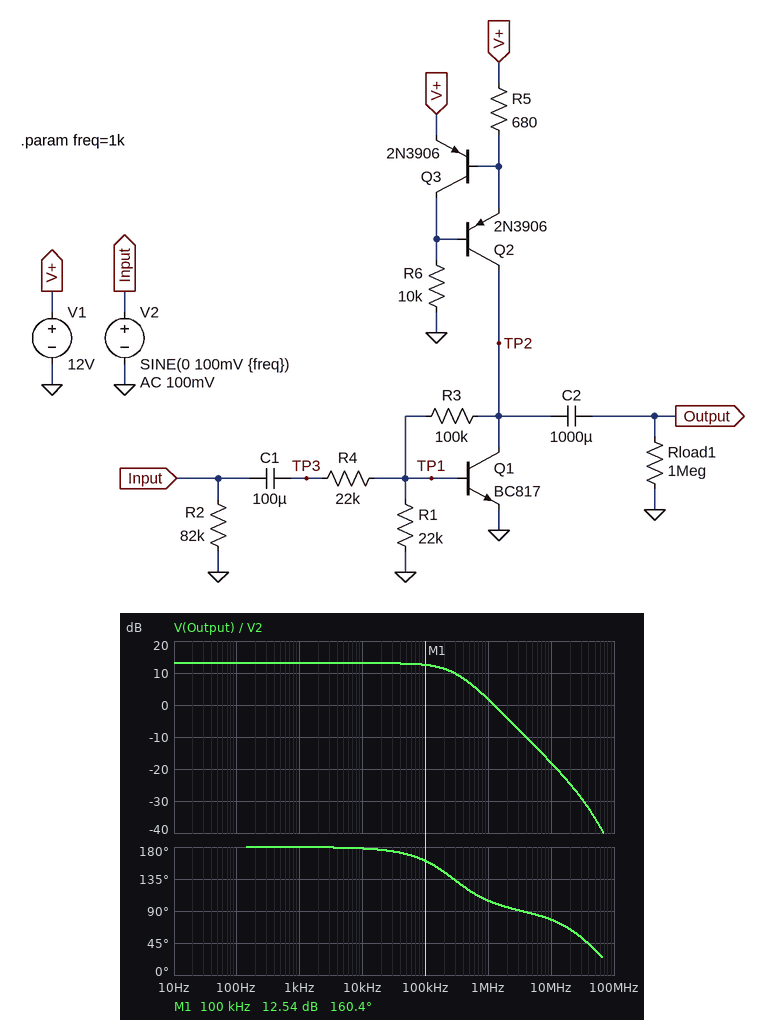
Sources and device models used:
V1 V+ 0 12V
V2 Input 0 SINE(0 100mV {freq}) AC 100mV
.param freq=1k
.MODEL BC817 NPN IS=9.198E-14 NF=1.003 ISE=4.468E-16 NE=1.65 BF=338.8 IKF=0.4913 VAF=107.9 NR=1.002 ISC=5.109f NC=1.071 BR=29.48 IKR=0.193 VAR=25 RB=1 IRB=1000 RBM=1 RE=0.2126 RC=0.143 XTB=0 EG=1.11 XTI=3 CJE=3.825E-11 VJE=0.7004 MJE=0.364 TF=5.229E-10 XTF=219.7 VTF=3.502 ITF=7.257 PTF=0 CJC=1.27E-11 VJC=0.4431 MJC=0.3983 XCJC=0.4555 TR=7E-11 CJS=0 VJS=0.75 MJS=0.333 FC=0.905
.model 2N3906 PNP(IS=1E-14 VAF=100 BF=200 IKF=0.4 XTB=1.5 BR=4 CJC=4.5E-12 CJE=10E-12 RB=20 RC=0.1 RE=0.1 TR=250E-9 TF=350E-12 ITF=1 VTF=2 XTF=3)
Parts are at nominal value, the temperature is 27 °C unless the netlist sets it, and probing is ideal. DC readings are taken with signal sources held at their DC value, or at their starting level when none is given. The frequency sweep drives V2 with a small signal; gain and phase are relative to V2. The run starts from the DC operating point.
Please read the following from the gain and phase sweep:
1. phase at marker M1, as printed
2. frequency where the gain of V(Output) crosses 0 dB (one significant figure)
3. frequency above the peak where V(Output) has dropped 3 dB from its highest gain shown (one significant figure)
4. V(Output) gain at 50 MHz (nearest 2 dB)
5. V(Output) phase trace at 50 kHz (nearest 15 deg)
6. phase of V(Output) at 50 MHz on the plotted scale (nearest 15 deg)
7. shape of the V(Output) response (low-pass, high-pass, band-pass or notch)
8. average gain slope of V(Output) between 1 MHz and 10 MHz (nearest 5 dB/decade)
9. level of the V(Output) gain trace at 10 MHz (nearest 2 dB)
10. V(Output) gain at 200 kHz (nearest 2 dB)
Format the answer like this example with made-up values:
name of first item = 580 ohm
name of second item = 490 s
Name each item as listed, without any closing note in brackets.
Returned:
phase at marker M1, as printed = 160.4 deg
frequency where the gain of V(Output) crosses 0 dB = 1 MHz
frequency above the peak where V(Output) has dropped 3 dB from its highest gain shown = 300 kHz
V(Output) gain at 50 MHz = -36 dB
V(Output) phase trace at 50 kHz = 165 deg
phase of V(Output) at 50 MHz on the plotted scale = 30 deg
shape of the V(Output) response = low-pass
average gain slope of V(Output) between 1 MHz and 10 MHz = -20 dB/decade
level of the V(Output) gain trace at 10 MHz = -18 dB
V(Output) gain at 200 kHz = 12 dB
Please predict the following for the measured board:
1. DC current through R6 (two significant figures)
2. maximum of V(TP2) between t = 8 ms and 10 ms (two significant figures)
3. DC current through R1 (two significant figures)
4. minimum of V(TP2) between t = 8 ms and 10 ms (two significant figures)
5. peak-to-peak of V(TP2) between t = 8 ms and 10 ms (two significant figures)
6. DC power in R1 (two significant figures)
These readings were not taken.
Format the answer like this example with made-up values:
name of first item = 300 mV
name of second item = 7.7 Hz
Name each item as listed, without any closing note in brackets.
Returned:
DC current through R6 = 1.1 mA
maximum of V(TP2) between t = 8 ms and 10 ms = 4.0 V
DC current through R1 = 27 µA
minimum of V(TP2) between t = 8 ms and 10 ms = 3.1 V
peak-to-peak of V(TP2) between t = 8 ms and 10 ms = 900 mV
DC power in R1 = 16 µW
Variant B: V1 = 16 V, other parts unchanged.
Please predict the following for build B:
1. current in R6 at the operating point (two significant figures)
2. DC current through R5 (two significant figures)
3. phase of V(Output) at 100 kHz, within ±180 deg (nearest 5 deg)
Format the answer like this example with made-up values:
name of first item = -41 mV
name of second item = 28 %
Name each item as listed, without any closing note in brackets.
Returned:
current in R6 at the operating point = 1.5 mA
DC current through R5 = 980 µA
phase of V(Output) at 100 kHz, within ±180 deg = 160 deg
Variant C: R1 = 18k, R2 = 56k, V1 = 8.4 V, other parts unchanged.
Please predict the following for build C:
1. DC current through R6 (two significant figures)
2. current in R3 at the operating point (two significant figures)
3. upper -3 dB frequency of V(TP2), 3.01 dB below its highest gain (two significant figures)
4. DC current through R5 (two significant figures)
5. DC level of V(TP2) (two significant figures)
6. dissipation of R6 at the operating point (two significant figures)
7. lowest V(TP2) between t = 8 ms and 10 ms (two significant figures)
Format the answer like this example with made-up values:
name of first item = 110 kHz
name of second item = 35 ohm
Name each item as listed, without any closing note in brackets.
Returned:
DC current through R6 = 710 µA
current in R3 at the operating point = 36 µA
upper -3 dB frequency of V(TP2), 3.01 dB below its highest gain = 300 kHz
DC current through R5 = 950 µA
DC level of V(TP2) = 4.2 V
dissipation of R6 at the operating point = 5.0 mW
lowest V(TP2) between t = 8 ms and 10 ms = 3.7 V
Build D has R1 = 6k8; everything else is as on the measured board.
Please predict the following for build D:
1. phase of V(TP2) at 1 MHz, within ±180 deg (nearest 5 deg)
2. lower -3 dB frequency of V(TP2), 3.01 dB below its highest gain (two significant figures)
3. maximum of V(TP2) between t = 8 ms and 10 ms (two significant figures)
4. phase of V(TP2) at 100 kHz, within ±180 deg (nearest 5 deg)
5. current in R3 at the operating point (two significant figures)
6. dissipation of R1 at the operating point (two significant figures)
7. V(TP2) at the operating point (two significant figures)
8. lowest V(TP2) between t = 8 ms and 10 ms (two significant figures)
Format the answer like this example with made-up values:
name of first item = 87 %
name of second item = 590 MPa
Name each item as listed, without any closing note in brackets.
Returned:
phase of V(TP2) at 1 MHz, within ±180 deg = 110 deg
lower -3 dB frequency of V(TP2), 3.01 dB below its highest gain = 72 mHz
maximum of V(TP2) between t = 8 ms and 10 ms = 10 V
phase of V(TP2) at 100 kHz, within ±180 deg = 165 deg
current in R3 at the operating point = 90 µA
dissipation of R1 at the operating point = 52 µW
V(TP2) at the operating point = 9.6 V
lowest V(TP2) between t = 8 ms and 10 ms = 9.1 V
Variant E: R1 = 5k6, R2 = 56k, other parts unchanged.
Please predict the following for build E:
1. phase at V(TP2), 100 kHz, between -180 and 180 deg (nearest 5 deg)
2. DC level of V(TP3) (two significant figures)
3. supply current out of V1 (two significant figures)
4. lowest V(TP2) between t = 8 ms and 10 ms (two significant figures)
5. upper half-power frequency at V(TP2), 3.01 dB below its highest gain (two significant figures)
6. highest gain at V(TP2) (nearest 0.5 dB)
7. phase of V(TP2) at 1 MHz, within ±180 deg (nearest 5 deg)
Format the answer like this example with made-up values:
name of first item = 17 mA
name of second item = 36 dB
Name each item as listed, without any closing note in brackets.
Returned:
phase at V(TP2), 100 kHz, between -180 and 180 deg = 145 deg
DC level of V(TP3) = 590 mV
supply current out of V1 = 1.9 mA
lowest V(TP2) between t = 8 ms and 10 ms = 11 V
upper half-power frequency at V(TP2), 3.01 dB below its highest gain = 170 kHz
highest gain at V(TP2) = -5.0 dB
phase of V(TP2) at 1 MHz, within ±180 deg = 85 deg
